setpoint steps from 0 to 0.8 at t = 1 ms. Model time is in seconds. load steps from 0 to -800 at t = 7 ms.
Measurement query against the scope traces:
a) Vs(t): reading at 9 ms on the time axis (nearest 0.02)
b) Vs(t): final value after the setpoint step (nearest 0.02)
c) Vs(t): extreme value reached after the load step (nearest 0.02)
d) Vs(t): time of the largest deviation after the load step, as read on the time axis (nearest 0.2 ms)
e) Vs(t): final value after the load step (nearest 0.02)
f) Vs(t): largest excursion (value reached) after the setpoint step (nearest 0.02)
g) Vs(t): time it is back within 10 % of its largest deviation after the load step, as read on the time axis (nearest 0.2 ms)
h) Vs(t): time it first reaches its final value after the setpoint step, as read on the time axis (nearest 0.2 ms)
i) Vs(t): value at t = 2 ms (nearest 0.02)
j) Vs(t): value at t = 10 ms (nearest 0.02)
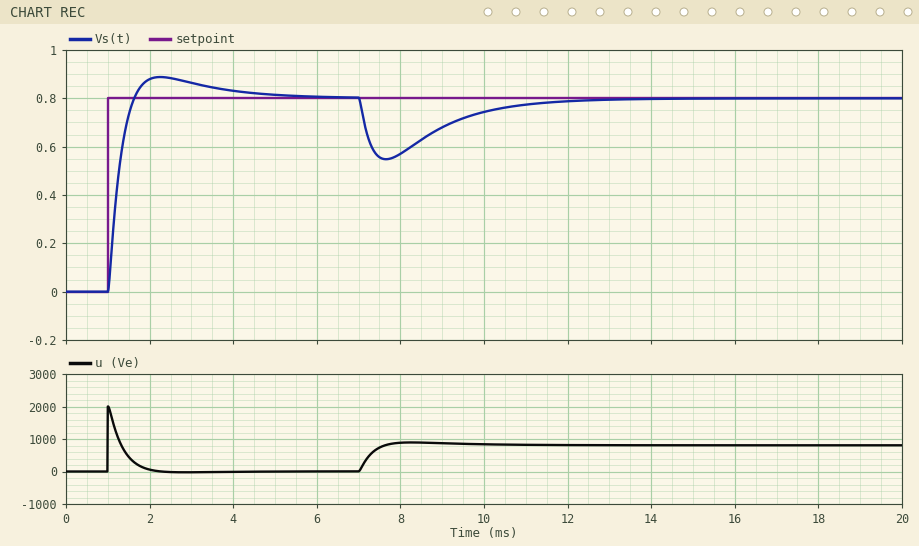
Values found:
0.68
0.80
0.54
7.6 ms
0.80
0.88
11.0 ms
1.6 ms
0.88
0.74
